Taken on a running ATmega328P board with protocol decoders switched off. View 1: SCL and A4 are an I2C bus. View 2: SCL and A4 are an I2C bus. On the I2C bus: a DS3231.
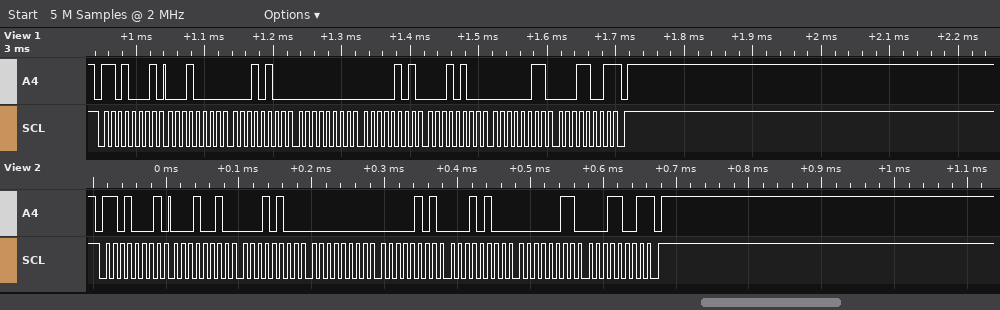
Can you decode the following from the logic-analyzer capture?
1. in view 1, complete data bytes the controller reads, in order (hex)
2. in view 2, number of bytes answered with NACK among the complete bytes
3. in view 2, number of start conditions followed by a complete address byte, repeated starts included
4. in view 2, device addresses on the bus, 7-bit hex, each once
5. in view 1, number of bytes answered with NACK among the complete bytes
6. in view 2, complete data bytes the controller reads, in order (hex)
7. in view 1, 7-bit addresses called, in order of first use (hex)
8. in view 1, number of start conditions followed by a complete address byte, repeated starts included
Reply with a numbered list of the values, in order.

1. 10 14 00 05 14 03 19
2. 1
3. 1
4. 0x68
5. 1
6. 12 14 00 05 14 03 19
7. 0x68
8. 1
